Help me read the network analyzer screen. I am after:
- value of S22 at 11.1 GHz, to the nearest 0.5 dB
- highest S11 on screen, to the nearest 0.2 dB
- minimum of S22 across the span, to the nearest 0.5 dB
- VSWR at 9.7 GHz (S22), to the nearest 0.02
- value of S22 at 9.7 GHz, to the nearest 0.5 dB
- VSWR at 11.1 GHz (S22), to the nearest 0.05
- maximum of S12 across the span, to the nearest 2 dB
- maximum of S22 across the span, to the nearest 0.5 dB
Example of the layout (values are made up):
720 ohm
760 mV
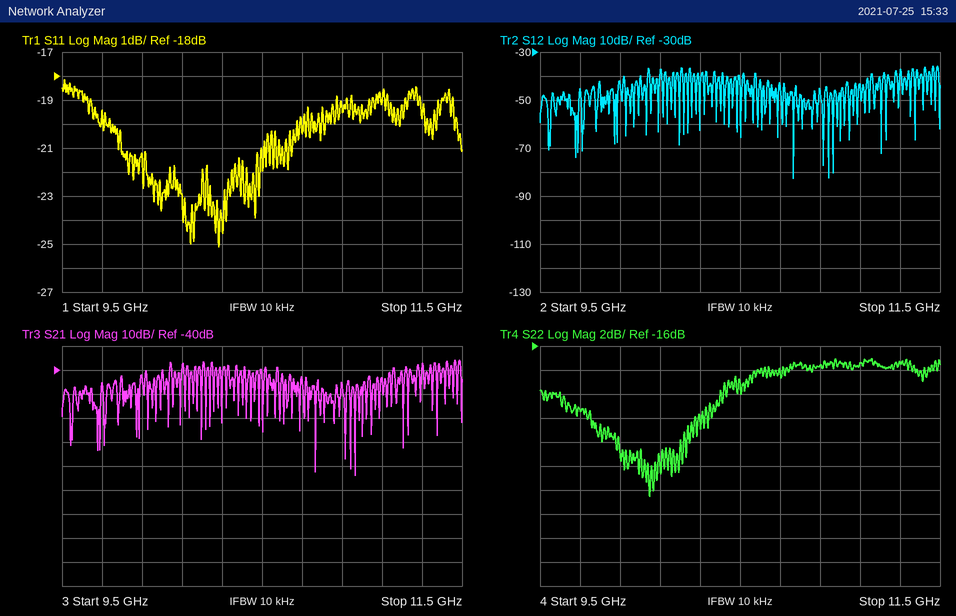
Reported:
-17.5 dB
-18.2 dB
-28.5 dB
1.18
-21.5 dB
1.30
-36 dB
-17.0 dB
